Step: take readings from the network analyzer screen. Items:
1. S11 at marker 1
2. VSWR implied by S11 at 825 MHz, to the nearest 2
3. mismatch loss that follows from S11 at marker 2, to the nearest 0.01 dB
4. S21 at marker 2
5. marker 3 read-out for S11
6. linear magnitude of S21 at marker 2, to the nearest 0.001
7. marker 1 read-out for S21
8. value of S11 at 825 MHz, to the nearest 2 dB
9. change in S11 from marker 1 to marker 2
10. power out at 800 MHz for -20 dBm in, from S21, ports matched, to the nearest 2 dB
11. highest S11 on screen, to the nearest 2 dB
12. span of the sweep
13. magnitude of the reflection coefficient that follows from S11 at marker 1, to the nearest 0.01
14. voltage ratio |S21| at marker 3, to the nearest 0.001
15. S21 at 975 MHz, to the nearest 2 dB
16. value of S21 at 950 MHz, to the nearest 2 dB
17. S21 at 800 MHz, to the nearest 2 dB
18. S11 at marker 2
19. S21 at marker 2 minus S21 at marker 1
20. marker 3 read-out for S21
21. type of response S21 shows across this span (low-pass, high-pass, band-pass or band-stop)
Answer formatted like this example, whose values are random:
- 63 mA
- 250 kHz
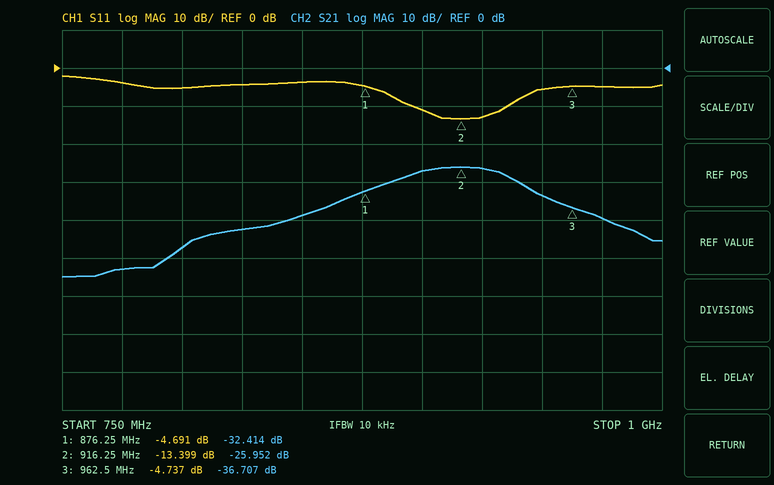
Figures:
- -4.691 dB
- 4
- 0.20 dB
- -25.952 dB
- -4.737 dB
- 0.050
- -32.414 dB
- -4 dB
- -8.708 dB
- -68 dBm
- -2 dB
- 250 MHz
- 0.58
- 0.015
- -40 dB
- -34 dB
- -48 dB
- -13.399 dB
- 6.462 dB
- -36.707 dB
- band-pass
